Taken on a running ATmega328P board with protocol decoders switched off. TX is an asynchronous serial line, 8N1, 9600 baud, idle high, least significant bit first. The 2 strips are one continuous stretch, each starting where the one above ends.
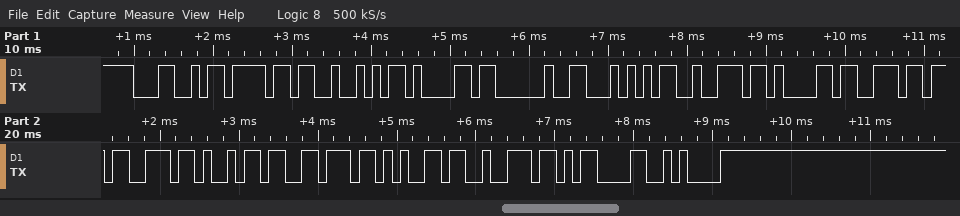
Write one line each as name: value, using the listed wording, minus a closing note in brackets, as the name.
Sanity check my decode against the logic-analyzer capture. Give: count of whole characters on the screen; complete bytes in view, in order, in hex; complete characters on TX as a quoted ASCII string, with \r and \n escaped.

count of whole characters on the screen: 16
complete bytes in view, in order, in hex: 4C 6F 52 61 20 54 72 61 6E 73 69 76 65 72 0D 0A
complete characters on TX as a quoted ASCII string, with \r and \n escaped: "LoRa Transiver\r\n"
